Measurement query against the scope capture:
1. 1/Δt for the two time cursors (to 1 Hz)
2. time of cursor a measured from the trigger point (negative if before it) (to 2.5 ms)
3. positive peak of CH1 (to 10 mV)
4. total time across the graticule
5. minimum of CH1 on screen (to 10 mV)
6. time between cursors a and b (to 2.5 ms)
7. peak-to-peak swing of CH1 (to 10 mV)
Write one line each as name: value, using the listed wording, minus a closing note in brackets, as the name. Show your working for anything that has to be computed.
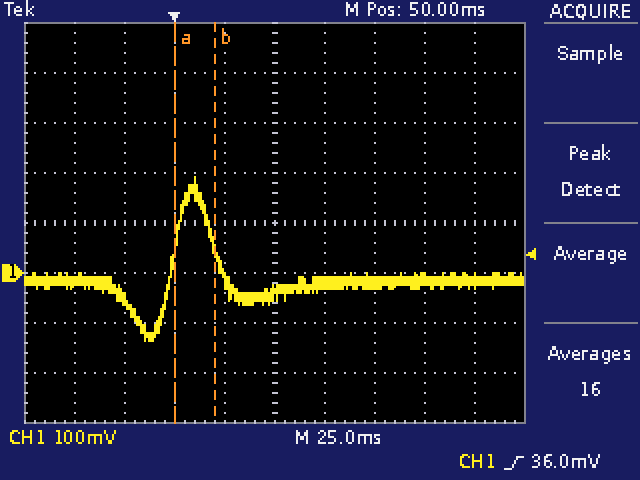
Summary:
1/Δt for the two time cursors: 1 / 20.0 ms ≈ 50 Hz
time of cursor a measured from the trigger point (negative if before it): 0.0 ms
positive peak of CH1: 190 mV
total time across the graticule: 250 ms
minimum of CH1 on screen: -140 mV
time between cursors a and b: 20.0 ms
peak-to-peak swing of CH1: 190 mV − (-140 mV) = 330 mV
